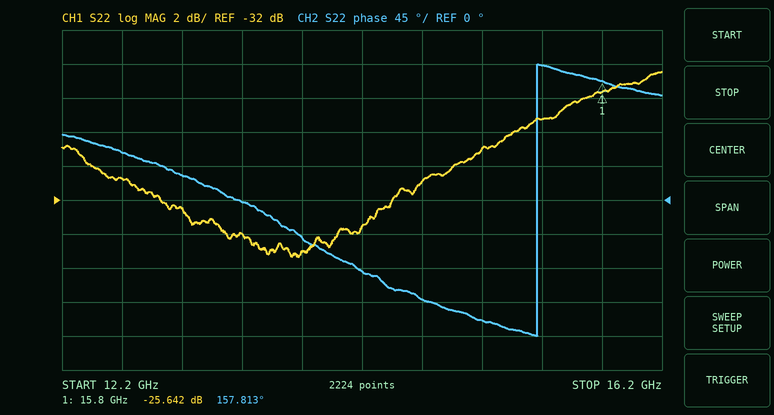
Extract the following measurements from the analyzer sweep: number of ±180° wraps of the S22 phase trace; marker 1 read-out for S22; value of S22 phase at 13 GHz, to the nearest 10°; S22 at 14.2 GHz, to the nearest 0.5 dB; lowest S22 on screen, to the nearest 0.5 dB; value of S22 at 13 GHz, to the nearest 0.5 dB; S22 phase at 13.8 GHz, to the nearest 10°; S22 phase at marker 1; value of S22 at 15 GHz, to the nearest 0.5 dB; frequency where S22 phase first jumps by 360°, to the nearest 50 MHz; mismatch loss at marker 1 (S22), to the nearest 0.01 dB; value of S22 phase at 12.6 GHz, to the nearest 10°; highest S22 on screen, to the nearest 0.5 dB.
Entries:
1
-25.642 dB
30°
-33.5 dB
-35.5 dB
-32.5 dB
-50°
157.813°
-29.0 dB
15.35 GHz
0.01 dB
60°
-24.5 dB
